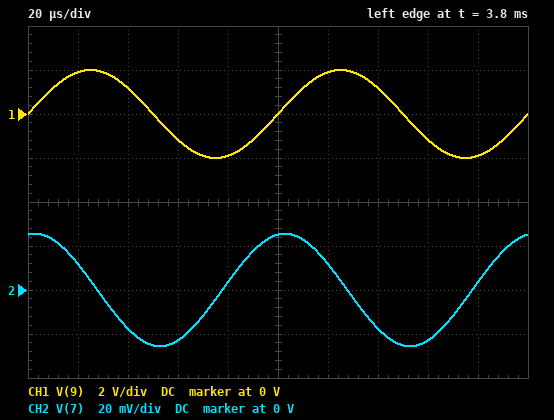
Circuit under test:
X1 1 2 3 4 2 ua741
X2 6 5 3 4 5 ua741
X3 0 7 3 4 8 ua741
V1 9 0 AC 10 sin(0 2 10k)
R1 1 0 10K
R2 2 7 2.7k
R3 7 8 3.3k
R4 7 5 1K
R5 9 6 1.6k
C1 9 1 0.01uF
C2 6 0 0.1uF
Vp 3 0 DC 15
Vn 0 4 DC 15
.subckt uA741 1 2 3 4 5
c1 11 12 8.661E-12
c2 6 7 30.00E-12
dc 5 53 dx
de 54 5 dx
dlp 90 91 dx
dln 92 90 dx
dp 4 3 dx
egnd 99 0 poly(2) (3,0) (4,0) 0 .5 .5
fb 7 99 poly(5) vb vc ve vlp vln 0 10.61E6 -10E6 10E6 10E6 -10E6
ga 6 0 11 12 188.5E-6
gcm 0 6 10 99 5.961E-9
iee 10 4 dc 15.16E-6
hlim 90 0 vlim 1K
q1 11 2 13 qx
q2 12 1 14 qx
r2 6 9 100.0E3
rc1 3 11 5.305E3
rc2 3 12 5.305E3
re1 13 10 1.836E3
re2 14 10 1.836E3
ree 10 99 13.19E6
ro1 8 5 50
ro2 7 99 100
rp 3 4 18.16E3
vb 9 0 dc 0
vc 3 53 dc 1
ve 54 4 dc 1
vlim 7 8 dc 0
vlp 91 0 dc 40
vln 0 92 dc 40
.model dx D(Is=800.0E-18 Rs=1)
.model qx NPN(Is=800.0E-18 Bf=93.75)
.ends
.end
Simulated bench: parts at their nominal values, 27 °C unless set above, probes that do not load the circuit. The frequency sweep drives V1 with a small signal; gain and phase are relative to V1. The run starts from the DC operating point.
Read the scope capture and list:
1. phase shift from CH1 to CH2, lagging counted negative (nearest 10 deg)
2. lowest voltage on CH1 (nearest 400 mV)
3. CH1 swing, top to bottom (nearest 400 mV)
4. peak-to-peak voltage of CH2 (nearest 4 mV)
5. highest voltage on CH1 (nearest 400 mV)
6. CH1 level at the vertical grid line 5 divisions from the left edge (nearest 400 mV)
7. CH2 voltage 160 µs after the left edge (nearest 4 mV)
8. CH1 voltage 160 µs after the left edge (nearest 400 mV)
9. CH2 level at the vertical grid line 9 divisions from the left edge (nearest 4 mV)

80 deg
-2.0 V
4.0 V
52 mV
2.0 V
0 V
-24 mV
-1.2 V
4 mV
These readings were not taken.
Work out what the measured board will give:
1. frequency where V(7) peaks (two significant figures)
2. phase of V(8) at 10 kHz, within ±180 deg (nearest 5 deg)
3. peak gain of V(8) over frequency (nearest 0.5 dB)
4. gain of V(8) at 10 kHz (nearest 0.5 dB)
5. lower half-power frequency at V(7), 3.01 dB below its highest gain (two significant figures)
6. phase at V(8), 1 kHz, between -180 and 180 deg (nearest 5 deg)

670 kHz
170 deg
10.5 dB
2.0 dB
180 kHz
150 deg
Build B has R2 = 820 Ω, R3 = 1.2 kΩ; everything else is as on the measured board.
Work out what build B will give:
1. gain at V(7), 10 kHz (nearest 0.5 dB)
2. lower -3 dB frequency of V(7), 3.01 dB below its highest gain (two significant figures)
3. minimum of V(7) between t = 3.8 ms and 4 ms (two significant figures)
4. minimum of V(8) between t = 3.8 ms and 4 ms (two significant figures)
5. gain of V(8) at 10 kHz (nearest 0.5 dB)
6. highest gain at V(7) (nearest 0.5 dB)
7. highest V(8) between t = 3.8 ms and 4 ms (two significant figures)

-36.5 dB
250 kHz
-31 mV
-2.9 V
3.0 dB
-7.5 dB
2.9 V
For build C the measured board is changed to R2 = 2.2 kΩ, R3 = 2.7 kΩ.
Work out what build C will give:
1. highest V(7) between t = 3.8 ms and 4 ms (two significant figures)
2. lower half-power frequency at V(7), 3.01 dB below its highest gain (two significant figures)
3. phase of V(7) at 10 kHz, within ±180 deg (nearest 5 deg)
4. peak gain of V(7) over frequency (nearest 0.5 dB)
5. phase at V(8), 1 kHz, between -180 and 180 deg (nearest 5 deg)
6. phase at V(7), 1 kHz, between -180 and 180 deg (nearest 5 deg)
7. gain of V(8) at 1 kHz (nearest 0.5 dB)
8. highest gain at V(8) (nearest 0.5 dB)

26 mV
200 kHz
85 deg
-11.5 dB
155 deg
65 deg
5.5 dB
8.5 dB
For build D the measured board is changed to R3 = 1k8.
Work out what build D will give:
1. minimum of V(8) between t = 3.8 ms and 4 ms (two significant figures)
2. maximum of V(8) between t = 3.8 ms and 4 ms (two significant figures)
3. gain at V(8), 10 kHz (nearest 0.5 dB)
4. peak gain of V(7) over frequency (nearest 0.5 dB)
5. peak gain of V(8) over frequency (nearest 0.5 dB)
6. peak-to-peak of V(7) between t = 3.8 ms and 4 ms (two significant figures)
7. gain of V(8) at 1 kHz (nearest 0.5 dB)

-1.3 V
1.3 V
-3.5 dB
-13.5 dB
5.0 dB
28 mV
2.0 dB
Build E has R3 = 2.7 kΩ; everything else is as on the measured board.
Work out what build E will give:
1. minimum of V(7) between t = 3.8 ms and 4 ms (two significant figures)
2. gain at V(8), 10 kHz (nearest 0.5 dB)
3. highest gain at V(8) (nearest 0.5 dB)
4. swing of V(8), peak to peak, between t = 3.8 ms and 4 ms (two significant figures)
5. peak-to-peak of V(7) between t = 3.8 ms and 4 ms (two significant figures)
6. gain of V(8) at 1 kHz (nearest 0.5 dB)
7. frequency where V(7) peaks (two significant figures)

-21 mV
0 dB
8.5 dB
4.0 V
42 mV
5.5 dB
700 kHz
